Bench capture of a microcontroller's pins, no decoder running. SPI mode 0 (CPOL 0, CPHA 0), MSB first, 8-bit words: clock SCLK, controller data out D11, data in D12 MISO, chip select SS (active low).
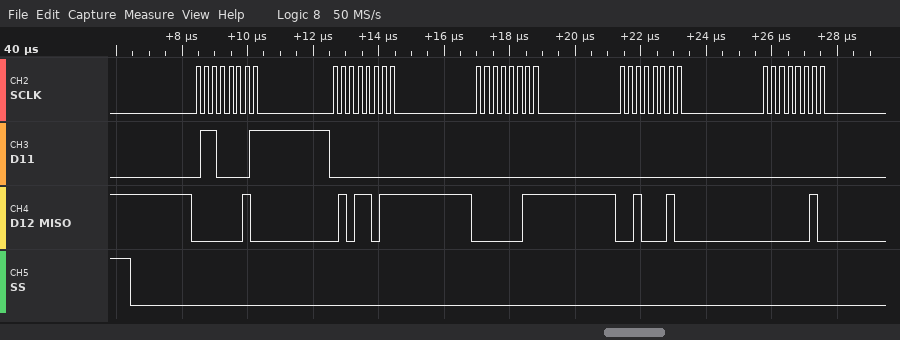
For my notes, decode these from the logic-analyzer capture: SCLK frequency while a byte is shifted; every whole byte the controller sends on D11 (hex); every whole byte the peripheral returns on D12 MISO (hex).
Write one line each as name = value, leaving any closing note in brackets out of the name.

SCLK frequency while a byte is shifted = 4 MHz
every whole byte the controller sends on D11 = 61 00 00 00 00
every whole byte the peripheral returns on D12 MISO = 02 5B 03 22 02
